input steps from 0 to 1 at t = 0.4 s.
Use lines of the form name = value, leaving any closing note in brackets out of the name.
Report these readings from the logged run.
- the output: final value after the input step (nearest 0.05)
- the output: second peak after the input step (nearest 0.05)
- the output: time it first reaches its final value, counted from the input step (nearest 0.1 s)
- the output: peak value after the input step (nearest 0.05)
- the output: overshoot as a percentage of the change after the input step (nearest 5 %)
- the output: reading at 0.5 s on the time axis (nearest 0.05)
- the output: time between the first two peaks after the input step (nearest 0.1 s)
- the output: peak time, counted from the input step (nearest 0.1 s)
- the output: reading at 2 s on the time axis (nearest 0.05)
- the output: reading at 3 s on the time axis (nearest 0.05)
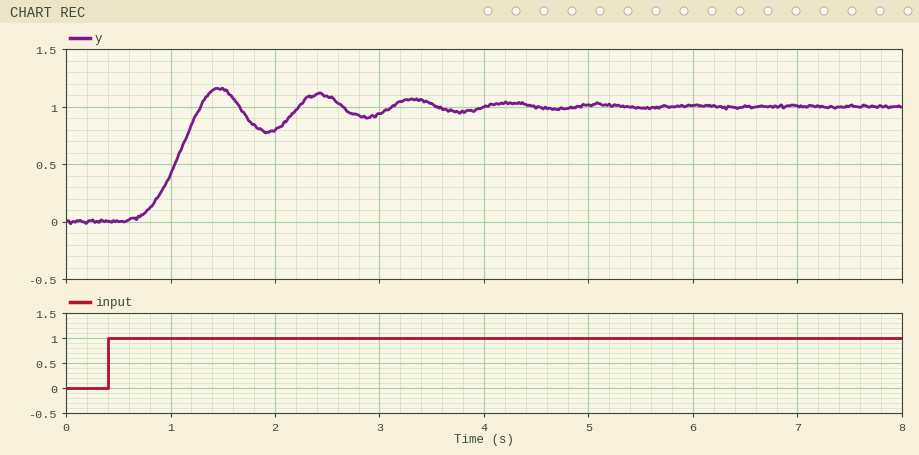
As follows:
the output: final value after the input step = 1.00
the output: second peak after the input step = 1.10
the output: time it first reaches its final value, counted from the input step = 0.9 s
the output: peak value after the input step = 1.15
the output: overshoot as a percentage of the change after the input step = 15 %
the output: reading at 0.5 s on the time axis = 0.00
the output: time between the first two peaks after the input step = 1.0 s
the output: peak time, counted from the input step = 1.1 s
the output: reading at 2 s on the time axis = 0.80
the output: reading at 3 s on the time axis = 0.95
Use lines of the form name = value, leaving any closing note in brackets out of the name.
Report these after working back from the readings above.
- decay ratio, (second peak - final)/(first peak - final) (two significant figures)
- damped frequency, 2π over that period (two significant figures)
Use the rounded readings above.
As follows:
decay ratio, (second peak - final)/(first peak - final) = 0.67
damped frequency, 2π over that period = 6.3 rad/s
